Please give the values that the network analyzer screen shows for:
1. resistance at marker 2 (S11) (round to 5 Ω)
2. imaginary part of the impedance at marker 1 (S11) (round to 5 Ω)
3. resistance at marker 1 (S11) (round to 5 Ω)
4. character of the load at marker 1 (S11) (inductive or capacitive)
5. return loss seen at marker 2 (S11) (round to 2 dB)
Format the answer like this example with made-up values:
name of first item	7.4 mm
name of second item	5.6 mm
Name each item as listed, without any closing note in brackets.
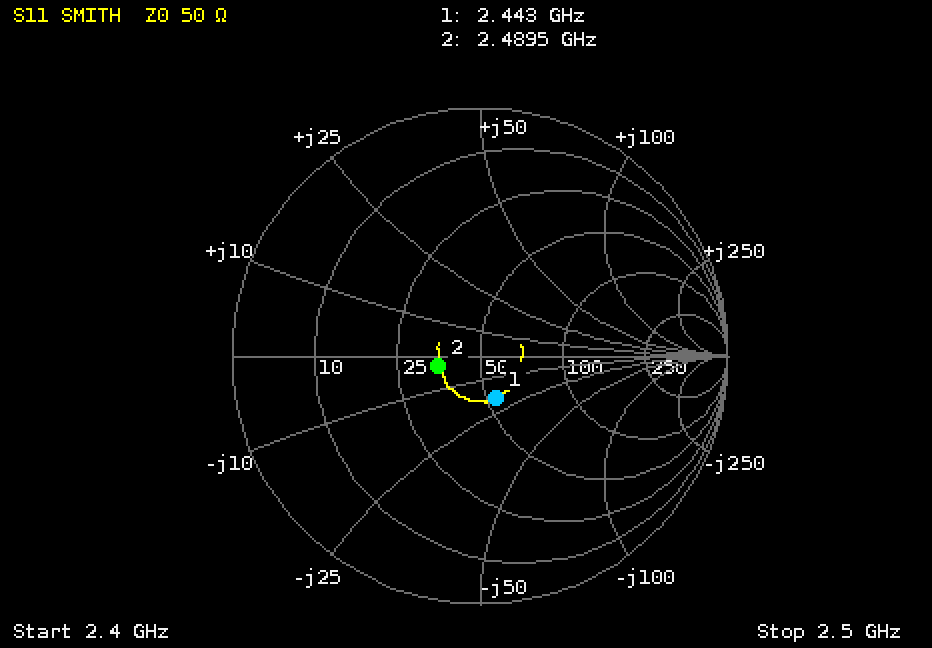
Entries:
resistance at marker 2 (S11)	35 Ω
imaginary part of the impedance at marker 1 (S11)	-20 Ω
resistance at marker 1 (S11)	55 Ω
character of the load at marker 1 (S11)	capacitive
return loss seen at marker 2 (S11)	16 dB
